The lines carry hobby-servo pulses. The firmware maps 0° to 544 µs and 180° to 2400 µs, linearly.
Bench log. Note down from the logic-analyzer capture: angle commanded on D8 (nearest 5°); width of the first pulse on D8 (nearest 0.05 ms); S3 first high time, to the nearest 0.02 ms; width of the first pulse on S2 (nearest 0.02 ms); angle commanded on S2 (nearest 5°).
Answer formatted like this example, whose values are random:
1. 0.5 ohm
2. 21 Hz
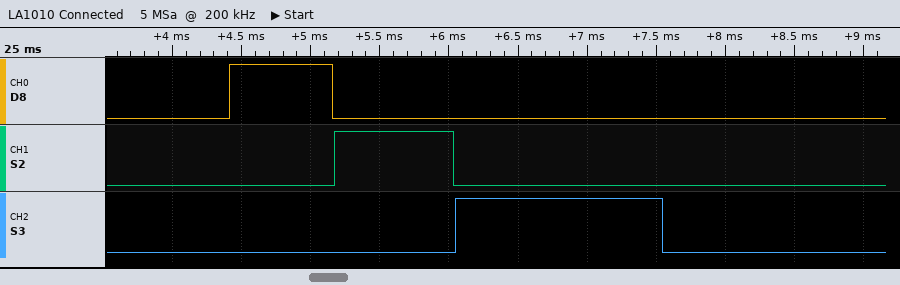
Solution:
1. 20°
2. 0.75 ms
3. 1.50 ms
4. 0.86 ms
5. 30°
